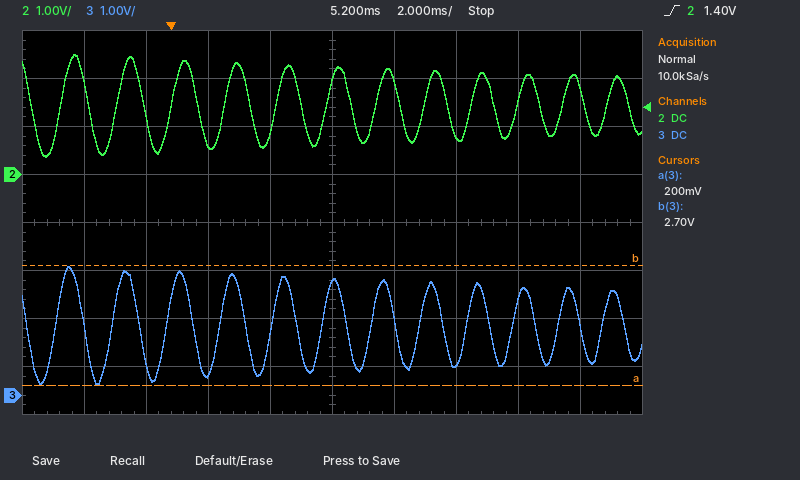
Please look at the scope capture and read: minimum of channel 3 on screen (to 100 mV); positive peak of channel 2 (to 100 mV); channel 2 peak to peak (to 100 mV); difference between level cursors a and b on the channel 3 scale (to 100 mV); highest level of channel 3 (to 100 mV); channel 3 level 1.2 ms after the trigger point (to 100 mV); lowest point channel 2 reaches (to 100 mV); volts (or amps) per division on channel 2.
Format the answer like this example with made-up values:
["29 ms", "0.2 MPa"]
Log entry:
["200 mV", "2.5 V", "2.1 V", "2.5 V", "2.7 V", "500 mV", "400 mV", "1 V"]
